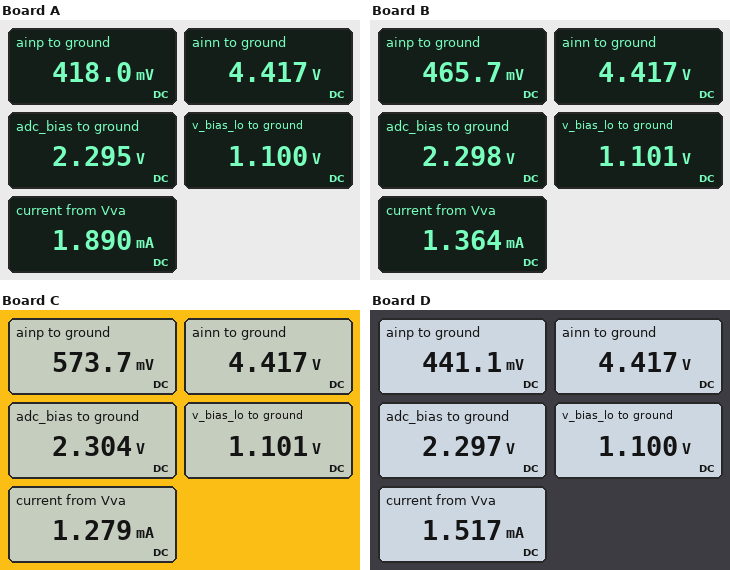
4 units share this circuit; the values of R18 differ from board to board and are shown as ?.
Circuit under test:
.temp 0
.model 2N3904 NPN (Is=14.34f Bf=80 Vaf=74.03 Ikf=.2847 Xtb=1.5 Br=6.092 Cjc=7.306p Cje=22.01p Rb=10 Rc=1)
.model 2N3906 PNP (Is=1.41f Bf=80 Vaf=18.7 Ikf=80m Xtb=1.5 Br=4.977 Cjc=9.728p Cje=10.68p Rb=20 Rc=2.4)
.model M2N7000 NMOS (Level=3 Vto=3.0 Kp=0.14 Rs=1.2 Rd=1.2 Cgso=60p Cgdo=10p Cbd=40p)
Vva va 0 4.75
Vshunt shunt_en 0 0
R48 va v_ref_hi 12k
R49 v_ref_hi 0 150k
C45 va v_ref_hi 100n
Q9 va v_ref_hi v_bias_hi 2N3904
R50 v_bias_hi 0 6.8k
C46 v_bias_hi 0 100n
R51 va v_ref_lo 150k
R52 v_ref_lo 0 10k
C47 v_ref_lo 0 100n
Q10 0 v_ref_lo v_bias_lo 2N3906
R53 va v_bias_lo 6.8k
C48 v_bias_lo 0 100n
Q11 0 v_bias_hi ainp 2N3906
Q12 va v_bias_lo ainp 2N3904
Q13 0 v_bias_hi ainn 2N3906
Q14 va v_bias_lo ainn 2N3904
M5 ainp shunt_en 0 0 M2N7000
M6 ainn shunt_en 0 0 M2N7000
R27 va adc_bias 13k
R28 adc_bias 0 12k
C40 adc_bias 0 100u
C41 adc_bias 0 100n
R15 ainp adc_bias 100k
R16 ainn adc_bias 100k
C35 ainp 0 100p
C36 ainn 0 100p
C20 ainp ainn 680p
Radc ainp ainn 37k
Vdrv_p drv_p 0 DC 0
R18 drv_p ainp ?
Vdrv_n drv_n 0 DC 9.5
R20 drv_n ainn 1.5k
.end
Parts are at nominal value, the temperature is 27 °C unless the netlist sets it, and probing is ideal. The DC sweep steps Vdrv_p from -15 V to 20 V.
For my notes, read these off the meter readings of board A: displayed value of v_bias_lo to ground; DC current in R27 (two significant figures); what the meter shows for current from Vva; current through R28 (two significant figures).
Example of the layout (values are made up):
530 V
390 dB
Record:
1.100 V
190 µA
1.890 mA
190 µA
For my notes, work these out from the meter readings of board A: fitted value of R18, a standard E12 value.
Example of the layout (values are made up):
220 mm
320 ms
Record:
560 Ω
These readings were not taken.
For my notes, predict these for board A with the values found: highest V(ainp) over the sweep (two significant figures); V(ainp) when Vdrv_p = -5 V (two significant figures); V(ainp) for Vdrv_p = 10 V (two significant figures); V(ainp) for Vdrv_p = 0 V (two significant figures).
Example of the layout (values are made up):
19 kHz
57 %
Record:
4.6 V
330 mV
4.5 V
420 mV
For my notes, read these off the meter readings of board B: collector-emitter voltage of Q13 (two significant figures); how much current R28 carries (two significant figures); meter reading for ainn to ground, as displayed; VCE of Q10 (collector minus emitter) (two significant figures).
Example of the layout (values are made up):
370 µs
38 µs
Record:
-4.4 V
190 µA
4.417 V
-1.1 V
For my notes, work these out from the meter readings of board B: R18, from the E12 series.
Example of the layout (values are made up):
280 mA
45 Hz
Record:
2.2 kΩ
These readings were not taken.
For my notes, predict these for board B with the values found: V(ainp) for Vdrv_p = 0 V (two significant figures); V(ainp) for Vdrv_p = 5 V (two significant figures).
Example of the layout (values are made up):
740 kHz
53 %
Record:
470 mV
4.4 V
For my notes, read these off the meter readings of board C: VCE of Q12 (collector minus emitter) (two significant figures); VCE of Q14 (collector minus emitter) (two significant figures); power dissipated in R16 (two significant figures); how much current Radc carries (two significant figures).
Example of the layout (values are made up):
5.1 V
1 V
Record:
4.2 V
330 mV
45 µW
100 µA
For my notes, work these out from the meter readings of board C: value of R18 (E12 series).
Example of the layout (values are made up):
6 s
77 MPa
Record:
4.7 kΩ
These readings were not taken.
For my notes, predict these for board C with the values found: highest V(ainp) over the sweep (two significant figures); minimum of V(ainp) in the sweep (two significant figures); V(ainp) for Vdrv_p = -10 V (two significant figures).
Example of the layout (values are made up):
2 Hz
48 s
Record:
4.4 V
370 mV
390 mV
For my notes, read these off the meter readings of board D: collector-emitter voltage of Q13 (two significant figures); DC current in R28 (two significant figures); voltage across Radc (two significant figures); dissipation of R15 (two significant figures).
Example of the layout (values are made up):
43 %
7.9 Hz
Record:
-4.4 V
190 µA
4.0 V
34 µW
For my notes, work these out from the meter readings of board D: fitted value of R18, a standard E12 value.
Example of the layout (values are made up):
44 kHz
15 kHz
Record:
1.2 kΩ
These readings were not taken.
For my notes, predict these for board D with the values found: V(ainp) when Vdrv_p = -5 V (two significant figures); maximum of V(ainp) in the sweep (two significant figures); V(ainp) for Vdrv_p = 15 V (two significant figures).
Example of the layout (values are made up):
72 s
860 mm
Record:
360 mV
4.5 V
4.5 V
